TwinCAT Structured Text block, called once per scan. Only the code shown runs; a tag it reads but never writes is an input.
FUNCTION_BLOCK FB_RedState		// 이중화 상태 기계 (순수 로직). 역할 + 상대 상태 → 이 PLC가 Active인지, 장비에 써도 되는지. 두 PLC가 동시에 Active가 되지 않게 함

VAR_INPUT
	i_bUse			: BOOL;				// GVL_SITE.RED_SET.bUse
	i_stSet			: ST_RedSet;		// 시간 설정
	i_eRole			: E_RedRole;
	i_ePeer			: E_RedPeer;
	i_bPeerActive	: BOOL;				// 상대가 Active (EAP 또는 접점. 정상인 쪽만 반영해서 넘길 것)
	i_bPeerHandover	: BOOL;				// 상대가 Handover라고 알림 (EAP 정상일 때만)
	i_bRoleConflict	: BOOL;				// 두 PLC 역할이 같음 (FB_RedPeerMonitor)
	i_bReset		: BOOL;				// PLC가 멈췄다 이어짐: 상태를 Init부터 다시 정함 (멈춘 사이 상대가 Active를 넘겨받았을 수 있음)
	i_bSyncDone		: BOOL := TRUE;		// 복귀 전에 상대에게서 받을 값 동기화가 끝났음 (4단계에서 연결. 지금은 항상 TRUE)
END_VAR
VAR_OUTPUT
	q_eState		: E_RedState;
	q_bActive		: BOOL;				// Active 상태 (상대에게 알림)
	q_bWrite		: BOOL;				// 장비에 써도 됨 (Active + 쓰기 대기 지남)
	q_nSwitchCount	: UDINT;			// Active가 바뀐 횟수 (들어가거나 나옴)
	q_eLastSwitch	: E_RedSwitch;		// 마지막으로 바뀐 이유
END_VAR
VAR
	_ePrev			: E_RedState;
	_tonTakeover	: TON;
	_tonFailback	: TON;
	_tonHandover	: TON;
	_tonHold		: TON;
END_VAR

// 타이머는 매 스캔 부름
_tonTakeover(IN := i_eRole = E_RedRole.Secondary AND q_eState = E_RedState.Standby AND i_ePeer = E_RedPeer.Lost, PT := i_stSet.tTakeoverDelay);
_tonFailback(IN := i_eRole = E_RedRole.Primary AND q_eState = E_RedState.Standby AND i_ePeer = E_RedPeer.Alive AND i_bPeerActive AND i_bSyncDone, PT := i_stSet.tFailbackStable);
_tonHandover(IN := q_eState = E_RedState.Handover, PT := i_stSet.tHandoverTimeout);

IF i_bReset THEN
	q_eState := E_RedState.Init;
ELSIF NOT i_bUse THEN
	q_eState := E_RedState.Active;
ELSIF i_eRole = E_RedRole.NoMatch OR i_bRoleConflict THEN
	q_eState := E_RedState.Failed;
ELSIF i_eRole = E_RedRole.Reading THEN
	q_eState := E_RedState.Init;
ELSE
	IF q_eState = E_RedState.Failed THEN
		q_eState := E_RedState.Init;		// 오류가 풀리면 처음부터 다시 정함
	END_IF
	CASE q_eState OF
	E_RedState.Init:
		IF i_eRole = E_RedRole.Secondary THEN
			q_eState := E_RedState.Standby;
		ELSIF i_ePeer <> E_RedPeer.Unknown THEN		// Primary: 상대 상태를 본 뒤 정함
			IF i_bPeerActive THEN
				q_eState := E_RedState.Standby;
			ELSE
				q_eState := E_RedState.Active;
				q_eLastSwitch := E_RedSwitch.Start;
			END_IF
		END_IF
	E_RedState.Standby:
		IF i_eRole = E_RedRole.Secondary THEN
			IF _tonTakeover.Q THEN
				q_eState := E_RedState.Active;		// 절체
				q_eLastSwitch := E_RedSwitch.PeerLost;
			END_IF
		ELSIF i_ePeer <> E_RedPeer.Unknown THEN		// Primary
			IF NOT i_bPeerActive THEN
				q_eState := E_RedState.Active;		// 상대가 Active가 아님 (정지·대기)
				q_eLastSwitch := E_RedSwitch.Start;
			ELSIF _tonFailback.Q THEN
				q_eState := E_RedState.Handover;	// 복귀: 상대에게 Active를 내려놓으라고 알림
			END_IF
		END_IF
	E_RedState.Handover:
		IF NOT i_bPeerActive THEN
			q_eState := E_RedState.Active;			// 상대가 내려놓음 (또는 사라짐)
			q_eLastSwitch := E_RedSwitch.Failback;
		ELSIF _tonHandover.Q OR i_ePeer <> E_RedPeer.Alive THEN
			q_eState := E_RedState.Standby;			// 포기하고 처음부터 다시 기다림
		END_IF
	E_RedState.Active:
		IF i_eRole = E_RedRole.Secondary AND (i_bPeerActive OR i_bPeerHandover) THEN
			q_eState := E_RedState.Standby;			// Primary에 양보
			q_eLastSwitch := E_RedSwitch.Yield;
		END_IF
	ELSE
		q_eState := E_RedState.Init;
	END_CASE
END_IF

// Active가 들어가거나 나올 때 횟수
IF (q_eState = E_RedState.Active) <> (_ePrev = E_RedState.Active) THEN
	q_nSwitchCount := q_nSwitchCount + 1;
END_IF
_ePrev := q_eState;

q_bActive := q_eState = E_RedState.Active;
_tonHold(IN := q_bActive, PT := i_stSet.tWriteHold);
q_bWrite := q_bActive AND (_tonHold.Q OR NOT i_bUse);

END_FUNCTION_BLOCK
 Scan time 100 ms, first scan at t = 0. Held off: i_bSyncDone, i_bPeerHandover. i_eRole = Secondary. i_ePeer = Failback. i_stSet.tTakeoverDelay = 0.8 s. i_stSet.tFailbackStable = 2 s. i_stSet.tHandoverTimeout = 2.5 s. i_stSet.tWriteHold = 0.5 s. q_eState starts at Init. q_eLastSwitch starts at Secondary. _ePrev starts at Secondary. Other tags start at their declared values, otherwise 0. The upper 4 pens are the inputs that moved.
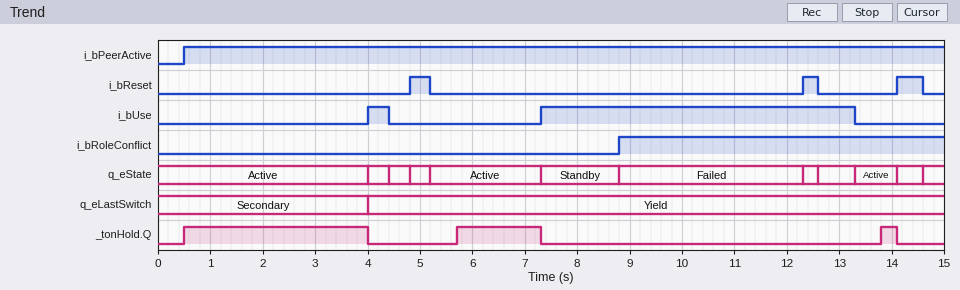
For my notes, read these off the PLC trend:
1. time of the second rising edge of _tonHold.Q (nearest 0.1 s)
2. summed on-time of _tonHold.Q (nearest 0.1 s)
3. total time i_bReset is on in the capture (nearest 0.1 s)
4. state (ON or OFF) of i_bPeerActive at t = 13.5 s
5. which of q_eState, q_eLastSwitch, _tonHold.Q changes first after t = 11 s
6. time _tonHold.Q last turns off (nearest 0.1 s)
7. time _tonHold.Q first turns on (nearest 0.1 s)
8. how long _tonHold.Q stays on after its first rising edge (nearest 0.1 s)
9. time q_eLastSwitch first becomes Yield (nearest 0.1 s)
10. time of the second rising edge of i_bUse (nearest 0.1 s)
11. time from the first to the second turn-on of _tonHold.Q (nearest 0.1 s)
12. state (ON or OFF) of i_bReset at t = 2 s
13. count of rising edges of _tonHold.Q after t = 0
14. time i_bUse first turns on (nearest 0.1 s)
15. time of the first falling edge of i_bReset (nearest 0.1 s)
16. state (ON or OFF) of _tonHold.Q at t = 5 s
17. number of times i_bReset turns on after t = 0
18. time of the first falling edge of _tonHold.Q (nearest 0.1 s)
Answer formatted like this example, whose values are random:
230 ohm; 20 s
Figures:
5.7 s; 5.4 s; 1.2 s; ON; q_eState; 14.1 s; 0.5 s; 3.5 s; 4.0 s; 7.3 s; 5.2 s; OFF; 3; 4.0 s; 5.2 s; OFF; 3; 4.0 s
